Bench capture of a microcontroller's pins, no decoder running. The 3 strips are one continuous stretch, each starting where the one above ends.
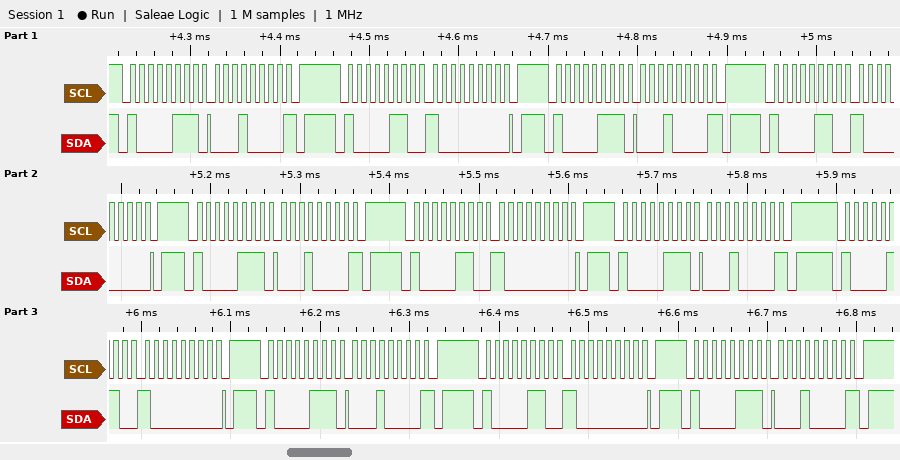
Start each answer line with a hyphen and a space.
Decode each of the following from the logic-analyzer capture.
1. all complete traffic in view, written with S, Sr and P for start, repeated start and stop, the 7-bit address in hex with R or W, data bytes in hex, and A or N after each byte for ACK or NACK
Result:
- S 43R A 10 N P S 43W A 80 A P S 43R A 10 N P S 43W A 80 A P S 43R A 10 N P S 43W A 80 A P S 43R A 10 N P S 43W A 80 A P S 43R A 10 N P S 43W A 80 A P S 43R A 10 N P
